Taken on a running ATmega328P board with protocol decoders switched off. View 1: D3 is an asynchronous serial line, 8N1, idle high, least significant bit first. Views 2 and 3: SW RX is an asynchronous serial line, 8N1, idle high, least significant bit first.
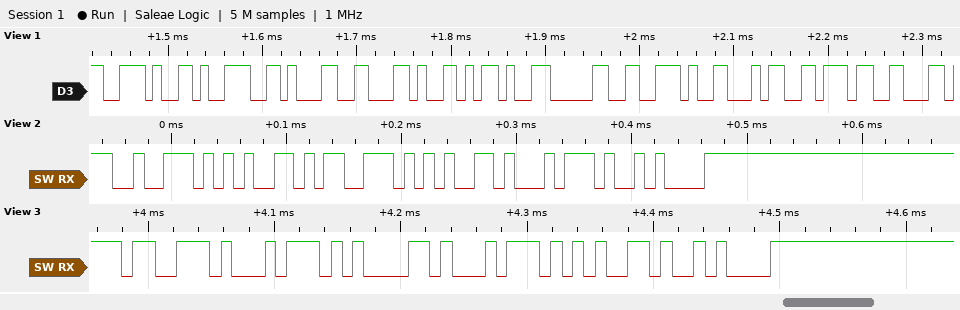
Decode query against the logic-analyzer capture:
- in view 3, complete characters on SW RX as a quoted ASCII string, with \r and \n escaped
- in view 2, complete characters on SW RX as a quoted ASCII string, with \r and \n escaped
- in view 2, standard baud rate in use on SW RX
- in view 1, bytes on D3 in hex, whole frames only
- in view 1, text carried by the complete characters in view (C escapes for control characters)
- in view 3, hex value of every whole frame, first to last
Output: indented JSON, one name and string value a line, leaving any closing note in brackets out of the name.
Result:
{
  "in view 3, complete characters on SW RX as a quoted ASCII string, with \\r and \\n escaped": "\"state\\n\"",
  "in view 2, complete characters on SW RX as a quoted ASCII string, with \\r and \\n escaped": "\"reset\\n\"",
  "in view 2, standard baud rate in use on SW RX": "115200 baud",
  "in view 1, bytes on D3 in hex, whole frames only": "0x2E 0x39 0x31 0x2C 0x2D 0x30 0x2E 0x34 0x37",
  "in view 1, text carried by the complete characters in view": "\".91,-0.47\"",
  "in view 3, hex value of every whole frame, first to last": "73 74 61 74 65 0A"
}
